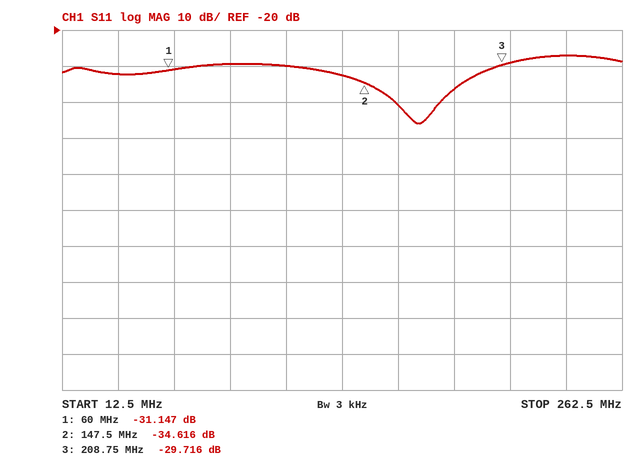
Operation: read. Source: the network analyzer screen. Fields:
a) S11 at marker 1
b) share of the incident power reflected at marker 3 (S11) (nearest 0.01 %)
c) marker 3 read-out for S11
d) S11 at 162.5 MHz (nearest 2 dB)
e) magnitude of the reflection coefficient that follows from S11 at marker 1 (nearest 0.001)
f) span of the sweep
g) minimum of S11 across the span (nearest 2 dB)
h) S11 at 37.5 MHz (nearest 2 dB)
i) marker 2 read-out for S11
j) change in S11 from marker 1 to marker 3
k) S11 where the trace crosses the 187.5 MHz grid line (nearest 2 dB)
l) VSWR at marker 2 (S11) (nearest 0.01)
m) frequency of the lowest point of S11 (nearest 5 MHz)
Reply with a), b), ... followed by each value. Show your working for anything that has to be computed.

a) -31.147 dB
b) 10^(-29.716/10) ≈ 0.11 %
c) -29.716 dB
d) -40 dB
e) 10^(-31.147/20) ≈ 0.028
f) 250 MHz
g) -46 dB
h) -32 dB
i) -34.616 dB
j) -29.716 − (-31.147) = 1.431 dB
k) -36 dB
l) (1 + 0.0186)/(1 − 0.0186) ≈ 1.04
m) 170 MHz
